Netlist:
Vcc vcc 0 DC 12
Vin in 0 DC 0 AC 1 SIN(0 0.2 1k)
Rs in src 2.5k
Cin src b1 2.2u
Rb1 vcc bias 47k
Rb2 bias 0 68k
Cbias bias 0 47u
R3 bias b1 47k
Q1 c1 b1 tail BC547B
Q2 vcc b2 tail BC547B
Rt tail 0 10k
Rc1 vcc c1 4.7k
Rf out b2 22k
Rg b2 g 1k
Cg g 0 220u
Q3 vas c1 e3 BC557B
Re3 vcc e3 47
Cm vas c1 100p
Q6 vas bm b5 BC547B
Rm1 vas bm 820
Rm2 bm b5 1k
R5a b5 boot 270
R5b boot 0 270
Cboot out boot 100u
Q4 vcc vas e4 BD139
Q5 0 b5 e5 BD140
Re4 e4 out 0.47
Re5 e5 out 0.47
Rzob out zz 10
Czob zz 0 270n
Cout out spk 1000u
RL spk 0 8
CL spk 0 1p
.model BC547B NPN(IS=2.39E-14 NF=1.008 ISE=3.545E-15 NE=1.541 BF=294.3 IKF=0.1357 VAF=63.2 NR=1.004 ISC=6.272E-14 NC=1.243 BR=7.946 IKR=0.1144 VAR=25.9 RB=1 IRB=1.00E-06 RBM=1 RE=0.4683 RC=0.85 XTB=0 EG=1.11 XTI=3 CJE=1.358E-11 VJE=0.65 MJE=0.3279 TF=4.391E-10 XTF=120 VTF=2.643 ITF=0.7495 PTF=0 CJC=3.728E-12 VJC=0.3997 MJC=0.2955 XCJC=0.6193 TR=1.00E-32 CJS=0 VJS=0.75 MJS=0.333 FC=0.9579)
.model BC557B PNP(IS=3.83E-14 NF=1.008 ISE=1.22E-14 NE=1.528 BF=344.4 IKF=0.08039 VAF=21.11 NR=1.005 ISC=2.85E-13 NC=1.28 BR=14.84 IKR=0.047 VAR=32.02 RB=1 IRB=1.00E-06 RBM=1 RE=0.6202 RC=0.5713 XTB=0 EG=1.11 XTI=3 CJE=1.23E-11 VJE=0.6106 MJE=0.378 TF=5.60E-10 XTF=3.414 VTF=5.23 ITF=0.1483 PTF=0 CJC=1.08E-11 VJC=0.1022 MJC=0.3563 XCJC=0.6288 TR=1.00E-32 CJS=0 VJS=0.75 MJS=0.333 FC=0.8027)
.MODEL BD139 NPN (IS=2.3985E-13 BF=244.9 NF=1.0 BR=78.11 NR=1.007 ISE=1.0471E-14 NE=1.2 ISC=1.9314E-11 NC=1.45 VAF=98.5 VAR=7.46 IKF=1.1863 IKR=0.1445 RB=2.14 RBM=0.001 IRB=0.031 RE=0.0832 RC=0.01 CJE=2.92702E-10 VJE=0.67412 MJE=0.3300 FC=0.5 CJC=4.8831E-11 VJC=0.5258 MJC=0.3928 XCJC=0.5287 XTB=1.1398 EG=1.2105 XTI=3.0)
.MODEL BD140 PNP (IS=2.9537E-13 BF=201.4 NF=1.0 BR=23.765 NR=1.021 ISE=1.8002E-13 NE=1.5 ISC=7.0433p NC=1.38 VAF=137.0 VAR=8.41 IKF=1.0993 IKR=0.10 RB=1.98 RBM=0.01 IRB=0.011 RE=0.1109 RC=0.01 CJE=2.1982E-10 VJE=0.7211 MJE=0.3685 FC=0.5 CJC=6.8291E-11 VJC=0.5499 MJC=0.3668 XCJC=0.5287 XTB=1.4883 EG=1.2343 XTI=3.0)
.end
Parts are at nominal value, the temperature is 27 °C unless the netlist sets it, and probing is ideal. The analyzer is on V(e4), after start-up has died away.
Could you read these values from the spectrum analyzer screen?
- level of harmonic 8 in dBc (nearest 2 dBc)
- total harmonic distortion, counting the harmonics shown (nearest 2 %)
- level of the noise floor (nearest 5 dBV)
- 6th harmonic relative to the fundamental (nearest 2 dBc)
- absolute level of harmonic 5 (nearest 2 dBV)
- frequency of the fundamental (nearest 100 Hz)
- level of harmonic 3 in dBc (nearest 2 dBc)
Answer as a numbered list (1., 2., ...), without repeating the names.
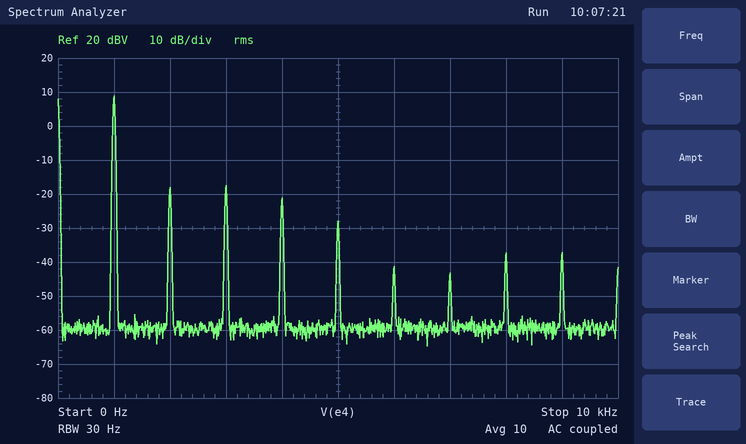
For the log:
1. -46 dBc
2. 8 %
3. -60 dBV
4. -50 dBc
5. -28 dBV
6. 1.0 kHz
7. -26 dBc
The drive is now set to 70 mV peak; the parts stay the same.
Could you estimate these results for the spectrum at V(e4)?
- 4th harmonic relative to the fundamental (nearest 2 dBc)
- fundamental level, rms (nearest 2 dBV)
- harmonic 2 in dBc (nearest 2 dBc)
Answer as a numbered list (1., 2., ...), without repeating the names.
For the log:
1. -56 dBc
2. 0 dBV
3. -38 dBc
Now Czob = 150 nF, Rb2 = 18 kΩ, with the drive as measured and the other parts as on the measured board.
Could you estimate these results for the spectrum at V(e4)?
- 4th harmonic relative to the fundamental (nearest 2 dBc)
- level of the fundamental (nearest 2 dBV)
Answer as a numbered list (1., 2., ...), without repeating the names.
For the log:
1. -34 dBc
2. 8 dBV
